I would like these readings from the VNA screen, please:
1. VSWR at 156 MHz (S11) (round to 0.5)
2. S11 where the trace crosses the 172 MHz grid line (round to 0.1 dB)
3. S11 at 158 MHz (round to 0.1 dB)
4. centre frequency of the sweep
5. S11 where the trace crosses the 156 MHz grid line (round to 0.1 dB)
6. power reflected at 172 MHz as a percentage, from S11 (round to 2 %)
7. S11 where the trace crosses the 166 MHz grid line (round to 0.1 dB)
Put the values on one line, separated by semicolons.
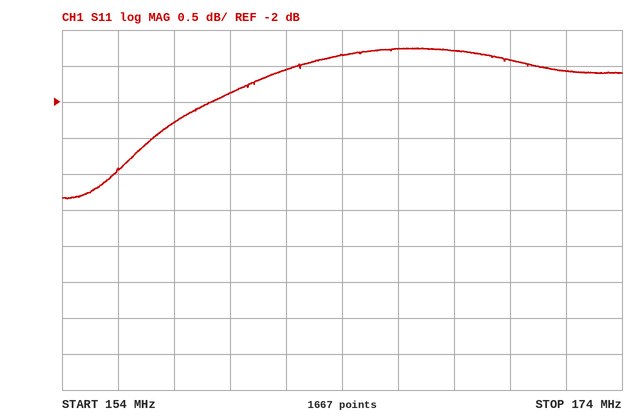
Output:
6.0; -1.6 dB; -2.3 dB; 164 MHz; -2.9 dB; 70 %; -1.3 dB
